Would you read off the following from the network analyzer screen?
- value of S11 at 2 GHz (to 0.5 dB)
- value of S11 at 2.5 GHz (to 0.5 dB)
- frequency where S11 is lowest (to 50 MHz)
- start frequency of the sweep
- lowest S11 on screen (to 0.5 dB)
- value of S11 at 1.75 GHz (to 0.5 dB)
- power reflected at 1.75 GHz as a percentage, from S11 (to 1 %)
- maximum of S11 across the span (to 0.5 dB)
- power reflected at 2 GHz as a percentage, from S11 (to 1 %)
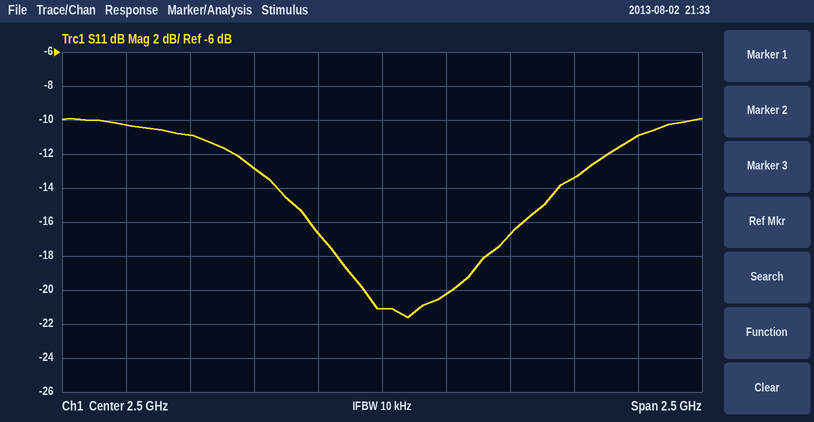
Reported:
-13.0 dB
-21.0 dB
2.60 GHz
1.25 GHz
-21.5 dB
-11.0 dB
8 %
-10.0 dB
5 %
